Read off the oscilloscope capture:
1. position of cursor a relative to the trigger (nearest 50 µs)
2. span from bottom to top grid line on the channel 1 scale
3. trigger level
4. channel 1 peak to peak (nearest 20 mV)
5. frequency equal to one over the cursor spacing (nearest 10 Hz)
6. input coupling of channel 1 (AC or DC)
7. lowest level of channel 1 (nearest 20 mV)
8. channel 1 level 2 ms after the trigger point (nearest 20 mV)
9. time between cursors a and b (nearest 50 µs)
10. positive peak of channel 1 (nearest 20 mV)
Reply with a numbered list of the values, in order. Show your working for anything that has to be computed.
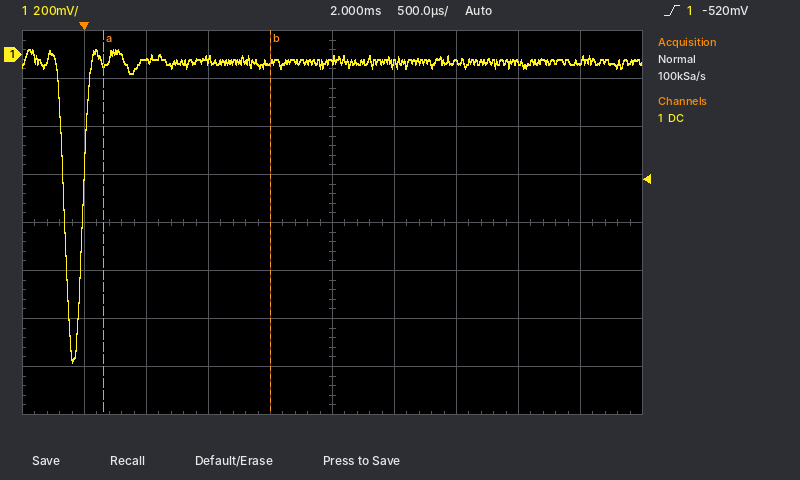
1. +150 µs
2. 1.6 V
3. -520 mV
4. 20 mV − (-1.28 V) = 1.30 V
5. 1 / 1.35 ms ≈ 740 Hz
6. DC
7. -1.28 V
8. -20 mV
9. 1.35 ms
10. 20 mV
